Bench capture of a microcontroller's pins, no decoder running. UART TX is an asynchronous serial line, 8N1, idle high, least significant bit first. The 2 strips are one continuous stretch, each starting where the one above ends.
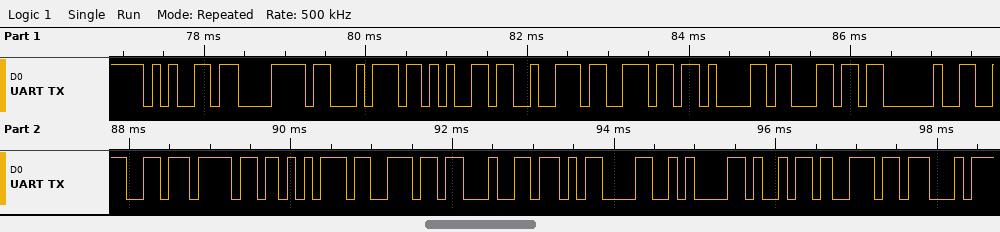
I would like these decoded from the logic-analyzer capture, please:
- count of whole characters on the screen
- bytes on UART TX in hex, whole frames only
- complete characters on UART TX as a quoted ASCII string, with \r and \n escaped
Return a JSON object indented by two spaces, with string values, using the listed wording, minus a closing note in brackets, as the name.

{
  "count of whole characters on the screen": "18",
  "bytes on UART TX in hex, whole frames only": "65 78 74 65 72 6E 61 6C 20 66 6F 75 6E 64 0D 0A 69 6E",
  "complete characters on UART TX as a quoted ASCII string, with \\r and \\n escaped": "\"external found\\r\\nin\""
}
